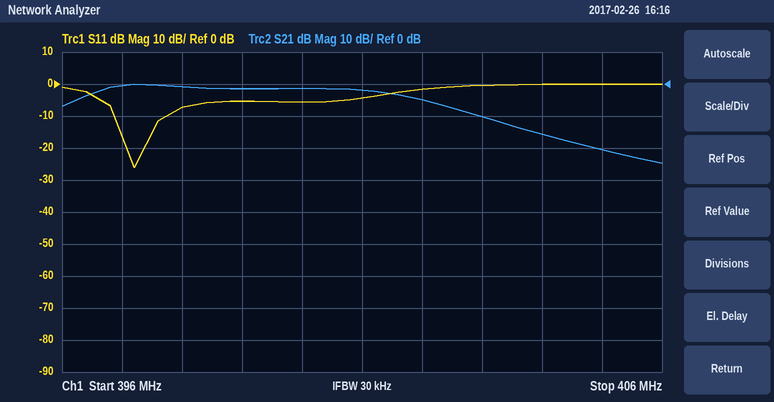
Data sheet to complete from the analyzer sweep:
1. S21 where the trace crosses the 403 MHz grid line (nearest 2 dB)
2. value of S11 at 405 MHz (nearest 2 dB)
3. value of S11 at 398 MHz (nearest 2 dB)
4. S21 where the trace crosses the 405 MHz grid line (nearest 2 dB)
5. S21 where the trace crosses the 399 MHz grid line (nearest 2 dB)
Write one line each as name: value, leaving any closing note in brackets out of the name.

S21 where the trace crosses the 403 MHz grid line: -10 dB
value of S11 at 405 MHz: 0 dB
value of S11 at 398 MHz: -8 dB
S21 where the trace crosses the 405 MHz grid line: -20 dB
S21 where the trace crosses the 399 MHz grid line: -2 dB
